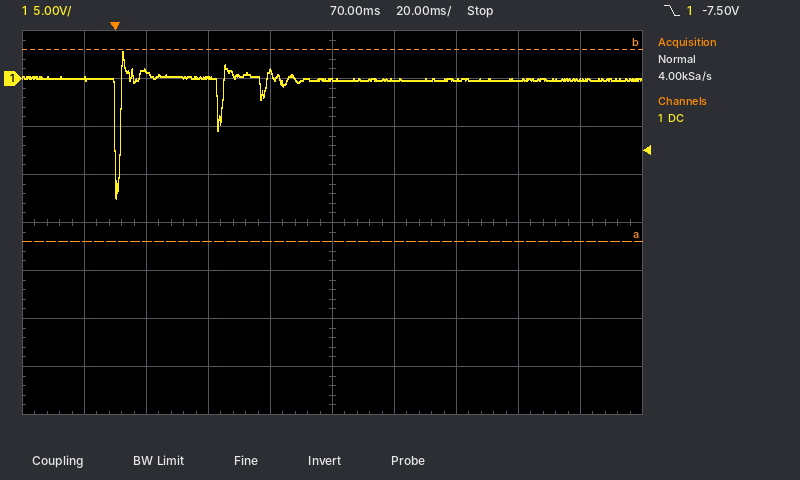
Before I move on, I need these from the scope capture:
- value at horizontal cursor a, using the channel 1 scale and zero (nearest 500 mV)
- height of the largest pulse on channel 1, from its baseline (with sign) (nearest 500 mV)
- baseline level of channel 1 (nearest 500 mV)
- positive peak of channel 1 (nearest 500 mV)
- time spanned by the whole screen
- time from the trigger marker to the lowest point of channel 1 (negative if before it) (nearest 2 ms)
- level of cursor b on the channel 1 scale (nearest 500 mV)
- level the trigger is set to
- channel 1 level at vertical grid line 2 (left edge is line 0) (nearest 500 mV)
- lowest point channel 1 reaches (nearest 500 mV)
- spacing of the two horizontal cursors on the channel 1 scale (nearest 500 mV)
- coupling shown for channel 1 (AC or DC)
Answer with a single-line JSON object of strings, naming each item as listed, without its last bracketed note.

{"value at horizontal cursor a, using the channel 1 scale and zero": "-17.0 V", "height of the largest pulse on channel 1, from its baseline (with sign)": "-12.5 V", "baseline level of channel 1": "0.0 V", "positive peak of channel 1": "3.0 V", "time spanned by the whole screen": "200 ms", "time from the trigger marker to the lowest point of channel 1 (negative if before it)": "0 ms", "level of cursor b on the channel 1 scale": "3.0 V", "level the trigger is set to": "-7.50 V", "channel 1 level at vertical grid line 2 (left edge is line 0)": "1.0 V", "lowest point channel 1 reaches": "-12.5 V", "spacing of the two horizontal cursors on the channel 1 scale": "20.0 V", "coupling shown for channel 1": "DC"}
